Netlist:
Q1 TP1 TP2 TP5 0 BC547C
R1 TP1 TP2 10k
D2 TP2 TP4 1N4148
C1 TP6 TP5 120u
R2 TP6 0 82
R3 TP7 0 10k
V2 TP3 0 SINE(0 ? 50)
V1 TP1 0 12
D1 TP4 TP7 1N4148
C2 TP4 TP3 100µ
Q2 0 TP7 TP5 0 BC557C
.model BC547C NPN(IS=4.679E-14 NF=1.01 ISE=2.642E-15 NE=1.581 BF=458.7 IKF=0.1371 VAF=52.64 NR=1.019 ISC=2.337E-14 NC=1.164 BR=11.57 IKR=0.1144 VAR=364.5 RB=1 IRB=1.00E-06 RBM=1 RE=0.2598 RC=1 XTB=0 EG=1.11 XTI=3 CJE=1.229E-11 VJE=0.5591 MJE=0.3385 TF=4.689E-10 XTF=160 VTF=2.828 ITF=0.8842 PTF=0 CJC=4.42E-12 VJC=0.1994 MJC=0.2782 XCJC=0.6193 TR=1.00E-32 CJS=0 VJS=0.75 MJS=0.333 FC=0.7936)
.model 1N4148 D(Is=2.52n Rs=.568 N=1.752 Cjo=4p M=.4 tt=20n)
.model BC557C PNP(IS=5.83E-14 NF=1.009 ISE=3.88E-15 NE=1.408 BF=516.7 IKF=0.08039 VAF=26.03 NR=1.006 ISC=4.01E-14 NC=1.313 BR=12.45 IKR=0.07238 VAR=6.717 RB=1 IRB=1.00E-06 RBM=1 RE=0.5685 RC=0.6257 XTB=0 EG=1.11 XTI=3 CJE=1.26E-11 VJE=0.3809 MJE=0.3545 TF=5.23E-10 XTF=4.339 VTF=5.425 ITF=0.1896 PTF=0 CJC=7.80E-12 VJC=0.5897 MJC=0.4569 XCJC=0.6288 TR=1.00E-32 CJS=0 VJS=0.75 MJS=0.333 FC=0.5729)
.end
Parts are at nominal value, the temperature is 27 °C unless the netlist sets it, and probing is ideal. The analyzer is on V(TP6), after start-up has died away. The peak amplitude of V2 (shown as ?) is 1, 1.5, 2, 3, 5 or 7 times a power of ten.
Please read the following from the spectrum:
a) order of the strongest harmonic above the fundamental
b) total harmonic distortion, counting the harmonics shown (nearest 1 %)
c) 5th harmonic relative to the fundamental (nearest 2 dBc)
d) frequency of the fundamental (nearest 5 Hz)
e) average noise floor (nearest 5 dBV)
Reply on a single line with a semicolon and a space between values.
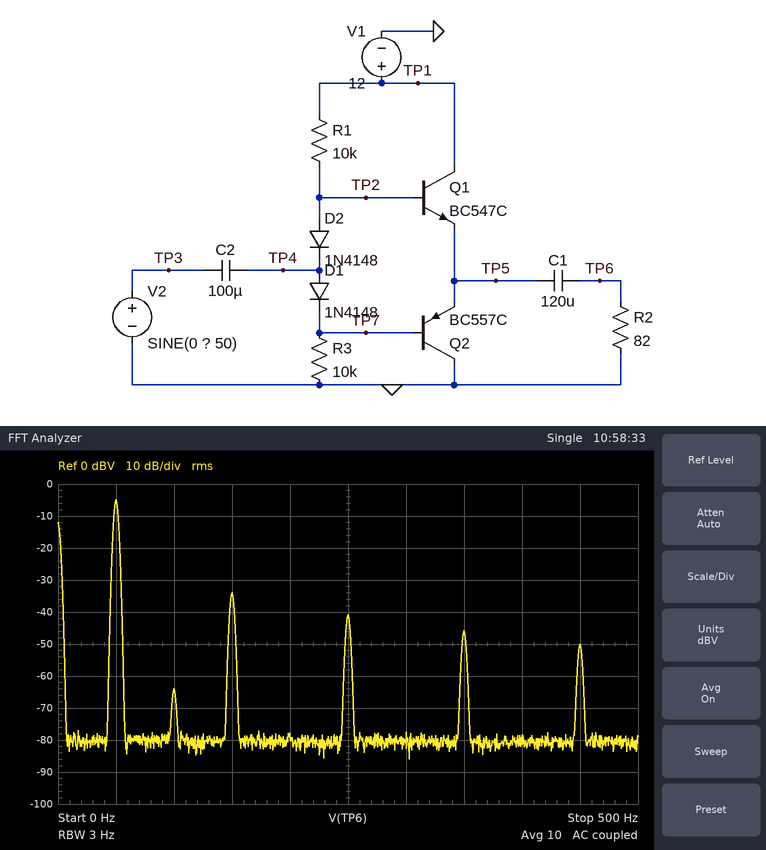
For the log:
3; 4 %; -36 dBc; 50 Hz; -80 dBV
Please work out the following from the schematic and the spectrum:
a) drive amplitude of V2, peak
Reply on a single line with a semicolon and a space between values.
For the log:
1 V
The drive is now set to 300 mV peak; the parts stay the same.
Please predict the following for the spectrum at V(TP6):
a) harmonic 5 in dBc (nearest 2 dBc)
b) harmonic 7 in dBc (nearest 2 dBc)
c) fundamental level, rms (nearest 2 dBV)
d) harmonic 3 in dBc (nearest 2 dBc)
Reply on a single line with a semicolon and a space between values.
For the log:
-34 dBc; -42 dBc; -18 dBV; -24 dBc
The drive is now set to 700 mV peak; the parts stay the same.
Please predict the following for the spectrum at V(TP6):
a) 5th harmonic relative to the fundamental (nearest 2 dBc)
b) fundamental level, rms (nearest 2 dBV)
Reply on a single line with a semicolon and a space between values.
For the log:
-34 dBc; -8 dBV
